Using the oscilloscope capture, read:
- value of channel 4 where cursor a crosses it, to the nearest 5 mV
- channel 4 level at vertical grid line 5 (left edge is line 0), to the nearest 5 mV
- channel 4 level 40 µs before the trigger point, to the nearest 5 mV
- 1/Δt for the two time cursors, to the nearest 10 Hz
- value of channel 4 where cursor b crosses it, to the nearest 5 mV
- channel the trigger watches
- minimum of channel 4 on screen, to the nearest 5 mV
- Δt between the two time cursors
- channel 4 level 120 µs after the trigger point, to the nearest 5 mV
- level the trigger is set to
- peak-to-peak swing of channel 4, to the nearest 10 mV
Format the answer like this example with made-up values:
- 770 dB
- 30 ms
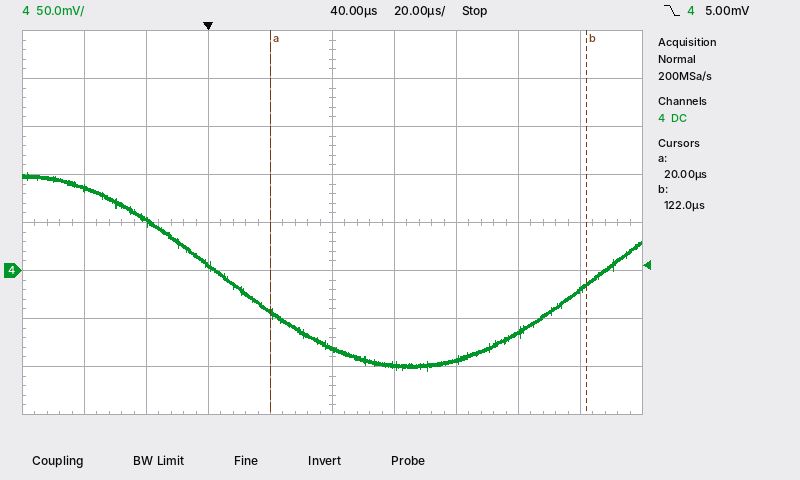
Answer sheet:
- -45 mV
- -80 mV
- 85 mV
- 9.80 kHz
- -15 mV
- channel 4
- -105 mV
- 102 µs
- -20 mV
- 5.00 mV
- 210 mV
